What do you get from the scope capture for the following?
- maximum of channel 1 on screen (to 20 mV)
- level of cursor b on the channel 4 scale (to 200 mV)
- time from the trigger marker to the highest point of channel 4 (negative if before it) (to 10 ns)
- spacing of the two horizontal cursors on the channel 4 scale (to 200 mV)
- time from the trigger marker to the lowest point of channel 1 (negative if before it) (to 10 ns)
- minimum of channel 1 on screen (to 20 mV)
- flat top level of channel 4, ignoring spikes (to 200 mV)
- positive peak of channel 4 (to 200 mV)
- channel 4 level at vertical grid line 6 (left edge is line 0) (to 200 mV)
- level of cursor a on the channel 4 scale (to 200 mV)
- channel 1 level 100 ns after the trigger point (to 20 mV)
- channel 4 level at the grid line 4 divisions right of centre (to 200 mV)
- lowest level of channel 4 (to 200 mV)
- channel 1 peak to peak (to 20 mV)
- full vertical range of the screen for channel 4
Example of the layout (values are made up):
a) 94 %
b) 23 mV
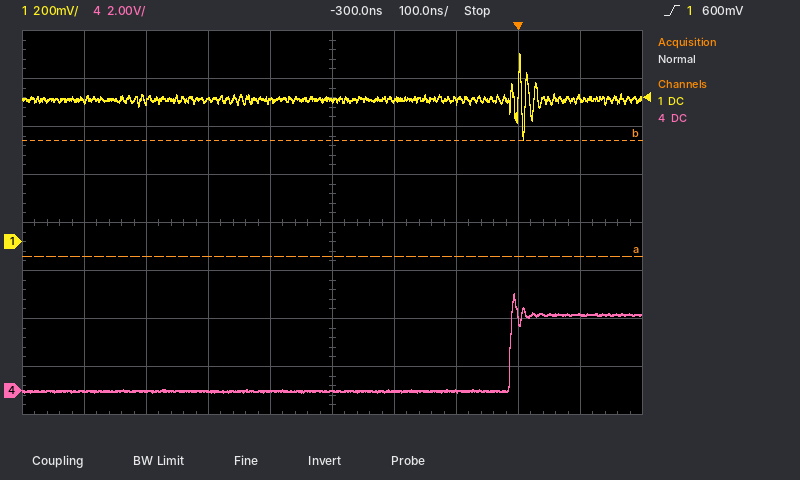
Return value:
a) 780 mV
b) 10.4 V
c) -10 ns
d) 4.8 V
e) +10 ns
f) 420 mV
g) 3.2 V
h) 4.0 V
i) 0.0 V
j) 5.6 V
k) 600 mV
l) 3.2 V
m) 0.0 V
n) 360 mV
o) 16 V
